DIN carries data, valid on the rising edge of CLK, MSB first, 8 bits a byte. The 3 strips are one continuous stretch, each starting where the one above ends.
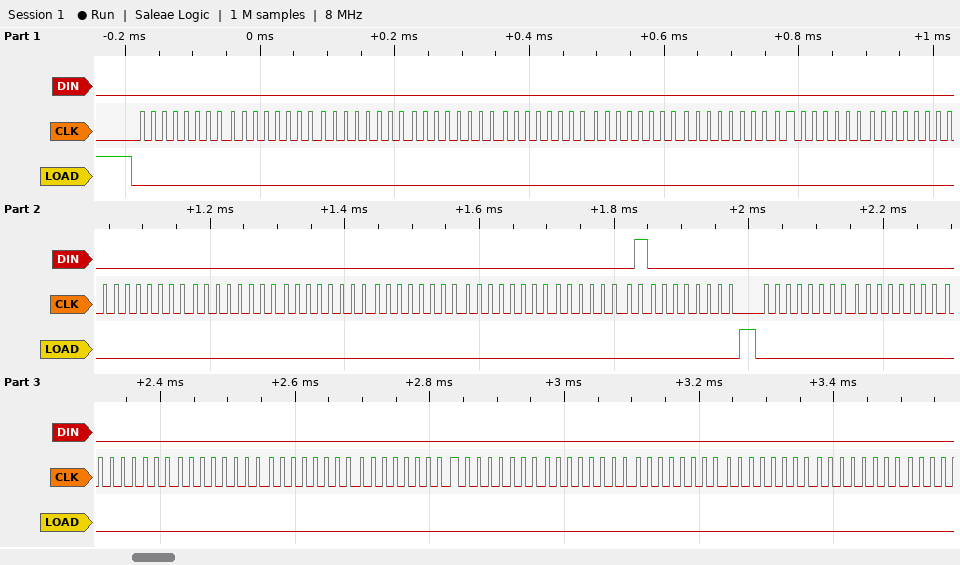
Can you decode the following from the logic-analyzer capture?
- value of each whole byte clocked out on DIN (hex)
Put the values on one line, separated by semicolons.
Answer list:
00 00 00 00 00 00 00 00 00 00 00 00 00 00 01 00 00 00 00 00 00 00 00 00 00 00 00
